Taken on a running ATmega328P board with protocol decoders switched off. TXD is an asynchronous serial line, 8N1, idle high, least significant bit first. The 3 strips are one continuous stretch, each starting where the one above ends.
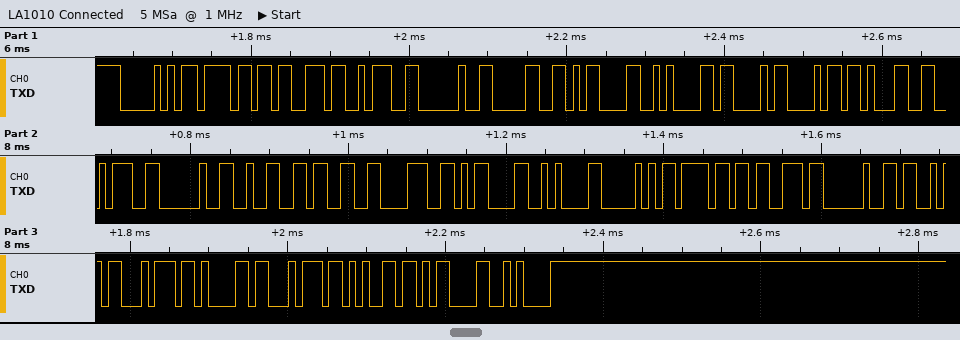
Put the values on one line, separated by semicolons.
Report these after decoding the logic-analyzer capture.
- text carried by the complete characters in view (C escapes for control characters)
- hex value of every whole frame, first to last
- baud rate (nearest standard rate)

"Pos: 0\r\nCh1: 238\r\nPos State\r\n"; 50 6F 73 3A 20 30 0D 0A 43 68 31 3A 20 32 33 38 0D 0A 50 6F 73 20 53 74 61 74 65 0D 0A; 115200 baud
